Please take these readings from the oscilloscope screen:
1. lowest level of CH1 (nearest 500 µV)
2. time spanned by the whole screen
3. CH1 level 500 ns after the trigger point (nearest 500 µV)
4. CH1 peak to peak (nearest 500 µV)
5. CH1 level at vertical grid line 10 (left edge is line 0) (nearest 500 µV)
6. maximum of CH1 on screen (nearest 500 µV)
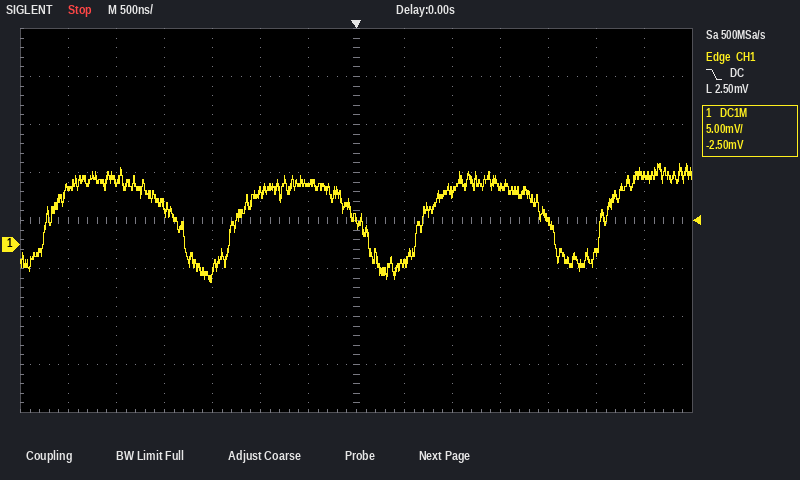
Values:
-4.0 mV
7 µs
-2.0 mV
12.5 mV
6.0 mV
8.5 mV
